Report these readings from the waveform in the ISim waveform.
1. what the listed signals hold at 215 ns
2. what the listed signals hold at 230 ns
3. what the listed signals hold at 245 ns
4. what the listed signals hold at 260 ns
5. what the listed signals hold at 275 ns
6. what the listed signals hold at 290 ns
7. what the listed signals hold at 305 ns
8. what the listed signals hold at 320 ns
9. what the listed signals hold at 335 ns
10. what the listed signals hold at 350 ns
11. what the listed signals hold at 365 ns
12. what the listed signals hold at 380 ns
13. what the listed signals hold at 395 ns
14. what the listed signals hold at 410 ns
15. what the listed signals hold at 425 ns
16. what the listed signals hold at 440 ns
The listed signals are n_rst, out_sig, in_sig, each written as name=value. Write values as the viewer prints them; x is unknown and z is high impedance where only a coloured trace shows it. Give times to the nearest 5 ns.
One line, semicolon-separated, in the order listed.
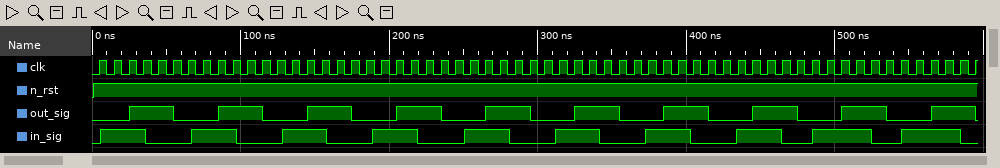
n_rst=1, out_sig=1, in_sig=1; n_rst=1, out_sig=1, in_sig=0; n_rst=1, out_sig=0, in_sig=0; n_rst=1, out_sig=0, in_sig=1; n_rst=1, out_sig=1, in_sig=1; n_rst=1, out_sig=1, in_sig=0; n_rst=1, out_sig=0, in_sig=0; n_rst=1, out_sig=0, in_sig=1; n_rst=1, out_sig=1, in_sig=1; n_rst=1, out_sig=1, in_sig=0; n_rst=1, out_sig=0, in_sig=0; n_rst=1, out_sig=0, in_sig=1; n_rst=1, out_sig=1, in_sig=1; n_rst=1, out_sig=1, in_sig=0; n_rst=1, out_sig=0, in_sig=0; n_rst=1, out_sig=0, in_sig=1
